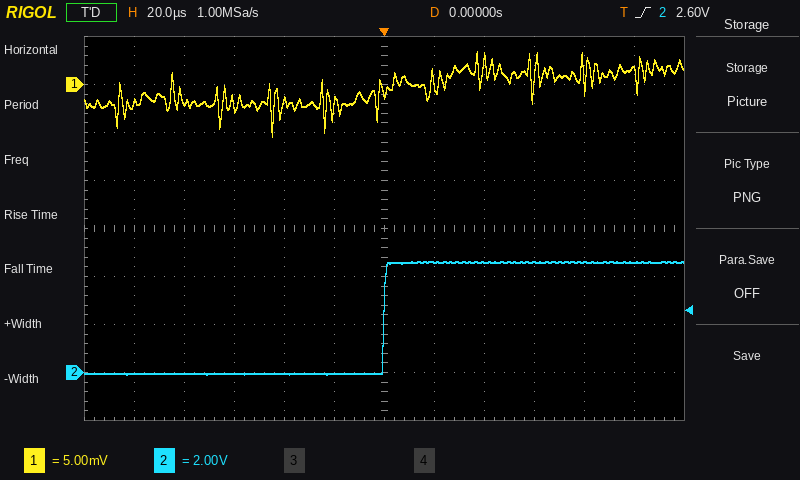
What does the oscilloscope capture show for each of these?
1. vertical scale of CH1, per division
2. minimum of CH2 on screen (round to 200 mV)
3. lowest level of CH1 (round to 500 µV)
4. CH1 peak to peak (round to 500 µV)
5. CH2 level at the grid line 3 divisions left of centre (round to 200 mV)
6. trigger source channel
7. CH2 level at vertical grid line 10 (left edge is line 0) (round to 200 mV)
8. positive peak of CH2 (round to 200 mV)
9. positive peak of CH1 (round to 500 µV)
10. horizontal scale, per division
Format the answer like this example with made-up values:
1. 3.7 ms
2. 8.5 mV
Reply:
1. 5 mV
2. 0.0 V
3. -5.5 mV
4. 9.0 mV
5. 0.0 V
6. CH2
7. 4.6 V
8. 4.6 V
9. 3.5 mV
10. 20 µs
